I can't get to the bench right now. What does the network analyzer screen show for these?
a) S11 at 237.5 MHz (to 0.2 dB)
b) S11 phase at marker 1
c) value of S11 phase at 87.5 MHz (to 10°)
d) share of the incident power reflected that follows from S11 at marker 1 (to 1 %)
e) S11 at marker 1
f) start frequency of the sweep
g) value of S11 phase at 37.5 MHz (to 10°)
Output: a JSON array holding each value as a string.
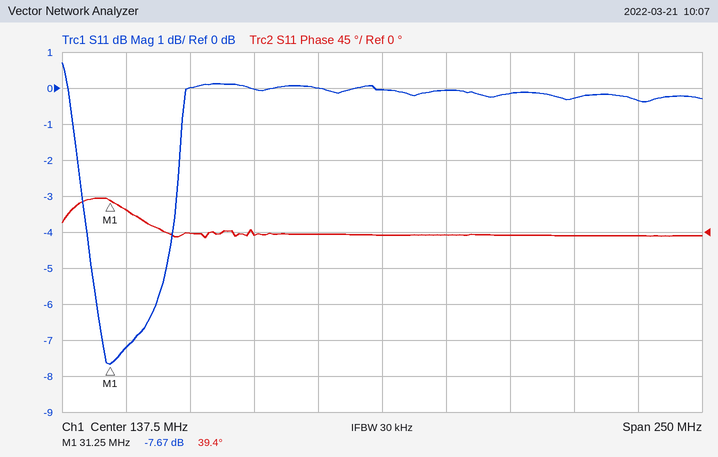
["-0.4 dB", "39.4°", "0°", "17 %", "-7.67 dB", "12.5 MHz", "30°"]
